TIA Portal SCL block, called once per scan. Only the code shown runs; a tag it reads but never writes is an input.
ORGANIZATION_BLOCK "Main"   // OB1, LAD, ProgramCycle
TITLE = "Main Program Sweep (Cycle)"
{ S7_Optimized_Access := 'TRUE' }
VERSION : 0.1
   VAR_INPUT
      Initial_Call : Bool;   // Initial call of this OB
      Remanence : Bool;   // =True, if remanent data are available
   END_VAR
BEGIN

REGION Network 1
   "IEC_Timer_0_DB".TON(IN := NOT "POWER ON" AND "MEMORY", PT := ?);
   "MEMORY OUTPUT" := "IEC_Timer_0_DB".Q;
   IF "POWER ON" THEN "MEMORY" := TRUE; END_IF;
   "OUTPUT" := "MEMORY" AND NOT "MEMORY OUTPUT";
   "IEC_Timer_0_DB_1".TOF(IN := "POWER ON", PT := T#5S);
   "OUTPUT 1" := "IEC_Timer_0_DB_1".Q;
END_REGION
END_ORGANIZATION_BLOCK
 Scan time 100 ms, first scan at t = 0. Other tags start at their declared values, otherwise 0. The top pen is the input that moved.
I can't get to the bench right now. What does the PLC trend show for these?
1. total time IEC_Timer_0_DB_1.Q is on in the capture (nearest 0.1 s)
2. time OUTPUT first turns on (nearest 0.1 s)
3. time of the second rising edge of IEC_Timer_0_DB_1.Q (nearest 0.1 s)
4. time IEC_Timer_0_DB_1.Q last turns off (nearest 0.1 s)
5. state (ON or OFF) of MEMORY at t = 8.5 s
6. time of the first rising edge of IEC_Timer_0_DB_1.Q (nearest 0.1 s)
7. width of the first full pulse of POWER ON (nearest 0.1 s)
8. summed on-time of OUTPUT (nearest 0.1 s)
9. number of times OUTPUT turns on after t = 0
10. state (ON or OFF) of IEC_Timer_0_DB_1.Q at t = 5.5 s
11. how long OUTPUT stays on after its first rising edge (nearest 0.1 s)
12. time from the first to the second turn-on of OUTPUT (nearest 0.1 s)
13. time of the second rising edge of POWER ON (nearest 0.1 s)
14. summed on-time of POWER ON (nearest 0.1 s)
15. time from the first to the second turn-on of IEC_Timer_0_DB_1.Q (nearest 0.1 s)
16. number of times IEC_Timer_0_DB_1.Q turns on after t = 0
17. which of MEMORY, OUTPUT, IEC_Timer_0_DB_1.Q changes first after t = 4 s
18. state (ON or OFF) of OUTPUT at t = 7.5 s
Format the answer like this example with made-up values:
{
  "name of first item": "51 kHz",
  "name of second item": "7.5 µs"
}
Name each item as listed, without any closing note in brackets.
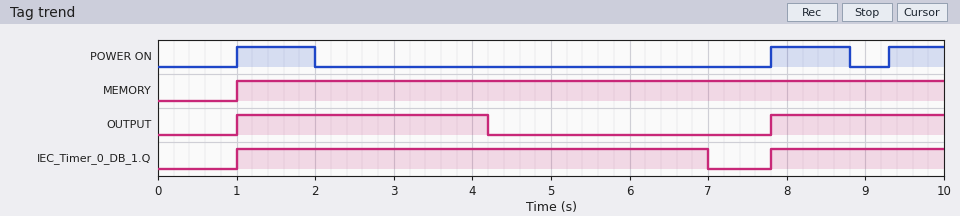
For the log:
{
  "total time IEC_Timer_0_DB_1.Q is on in the capture": "8.2 s",
  "time OUTPUT first turns on": "1.0 s",
  "time of the second rising edge of IEC_Timer_0_DB_1.Q": "7.8 s",
  "time IEC_Timer_0_DB_1.Q last turns off": "7.0 s",
  "state (ON or OFF) of MEMORY at t = 8.5 s": "ON",
  "time of the first rising edge of IEC_Timer_0_DB_1.Q": "1.0 s",
  "width of the first full pulse of POWER ON": "1.0 s",
  "summed on-time of OUTPUT": "5.4 s",
  "number of times OUTPUT turns on after t = 0": "2",
  "state (ON or OFF) of IEC_Timer_0_DB_1.Q at t = 5.5 s": "ON",
  "how long OUTPUT stays on after its first rising edge": "3.2 s",
  "time from the first to the second turn-on of OUTPUT": "6.8 s",
  "time of the second rising edge of POWER ON": "7.8 s",
  "summed on-time of POWER ON": "2.7 s",
  "time from the first to the second turn-on of IEC_Timer_0_DB_1.Q": "6.8 s",
  "number of times IEC_Timer_0_DB_1.Q turns on after t = 0": "2",
  "which of MEMORY, OUTPUT, IEC_Timer_0_DB_1.Q changes first after t = 4 s": "OUTPUT",
  "state (ON or OFF) of OUTPUT at t = 7.5 s": "OFF"
}
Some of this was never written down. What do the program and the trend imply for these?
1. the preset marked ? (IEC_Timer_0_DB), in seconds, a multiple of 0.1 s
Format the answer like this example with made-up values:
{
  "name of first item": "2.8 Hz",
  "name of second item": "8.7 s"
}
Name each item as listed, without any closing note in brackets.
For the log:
{
  "the preset marked ? (IEC_Timer_0_DB), in seconds, a multiple of 0.1 s": "2.2 s"
}
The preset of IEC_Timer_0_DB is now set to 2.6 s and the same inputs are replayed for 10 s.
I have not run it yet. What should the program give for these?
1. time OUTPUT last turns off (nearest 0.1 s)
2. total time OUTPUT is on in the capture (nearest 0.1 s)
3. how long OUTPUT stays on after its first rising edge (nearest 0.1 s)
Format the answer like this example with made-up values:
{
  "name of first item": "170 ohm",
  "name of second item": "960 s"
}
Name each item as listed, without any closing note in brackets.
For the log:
{
  "time OUTPUT last turns off": "4.6 s",
  "total time OUTPUT is on in the capture": "5.8 s",
  "how long OUTPUT stays on after its first rising edge": "3.6 s"
}
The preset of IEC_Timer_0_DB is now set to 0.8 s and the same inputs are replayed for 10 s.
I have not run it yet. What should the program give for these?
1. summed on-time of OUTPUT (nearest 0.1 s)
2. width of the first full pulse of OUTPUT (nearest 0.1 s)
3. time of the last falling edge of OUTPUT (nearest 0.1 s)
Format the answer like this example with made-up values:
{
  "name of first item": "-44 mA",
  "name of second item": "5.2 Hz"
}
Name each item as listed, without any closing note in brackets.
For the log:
{
  "summed on-time of OUTPUT": "4.0 s",
  "width of the first full pulse of OUTPUT": "1.8 s",
  "time of the last falling edge of OUTPUT": "2.8 s"
}
